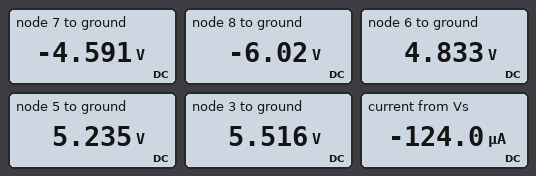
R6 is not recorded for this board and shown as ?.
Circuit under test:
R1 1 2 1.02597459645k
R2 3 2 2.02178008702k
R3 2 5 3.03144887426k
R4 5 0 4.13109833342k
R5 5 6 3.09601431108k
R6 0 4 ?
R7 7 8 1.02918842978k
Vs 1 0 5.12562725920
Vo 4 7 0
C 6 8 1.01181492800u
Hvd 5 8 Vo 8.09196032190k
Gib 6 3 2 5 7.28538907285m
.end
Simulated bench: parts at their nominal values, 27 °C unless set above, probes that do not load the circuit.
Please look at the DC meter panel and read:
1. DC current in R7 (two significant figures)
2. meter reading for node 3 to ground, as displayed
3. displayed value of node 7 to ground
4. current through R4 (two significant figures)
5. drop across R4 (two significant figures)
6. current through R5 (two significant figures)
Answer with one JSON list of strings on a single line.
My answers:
["1.4 mA", "5.516 V", "-4.591 V", "1.3 mA", "5.2 V", "130 µA"]
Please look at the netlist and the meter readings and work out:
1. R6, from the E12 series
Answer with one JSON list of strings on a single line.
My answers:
["3.3 kΩ"]
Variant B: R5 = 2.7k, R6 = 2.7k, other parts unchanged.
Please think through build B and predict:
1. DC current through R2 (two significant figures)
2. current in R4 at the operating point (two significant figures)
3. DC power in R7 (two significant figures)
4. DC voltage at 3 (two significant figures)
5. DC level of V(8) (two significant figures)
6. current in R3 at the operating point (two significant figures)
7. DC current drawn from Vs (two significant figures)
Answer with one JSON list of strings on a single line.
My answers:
["68 µA", "1.2 mA", "1.4 mW", "4.9 V", "-4.3 V", "3.1 µA", "65 µA"]
